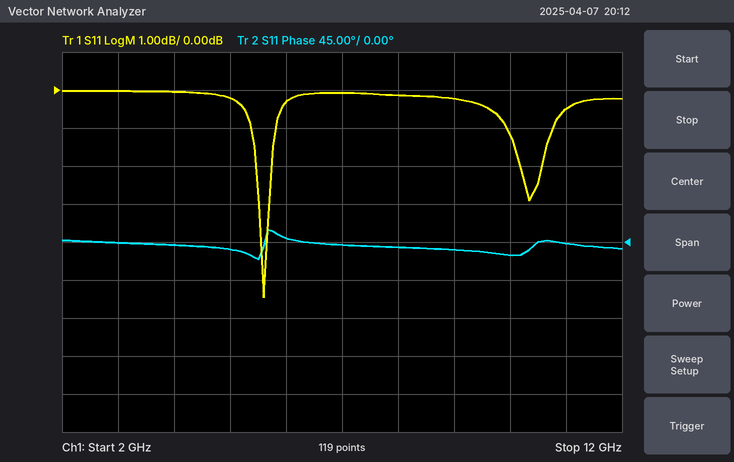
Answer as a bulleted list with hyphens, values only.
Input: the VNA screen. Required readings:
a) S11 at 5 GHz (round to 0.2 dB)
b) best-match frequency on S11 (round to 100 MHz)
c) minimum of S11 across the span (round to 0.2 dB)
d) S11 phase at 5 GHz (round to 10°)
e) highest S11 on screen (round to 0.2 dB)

- -0.2 dB
- 5.6 GHz
- -5.4 dB
- -10°
- 0.0 dB
